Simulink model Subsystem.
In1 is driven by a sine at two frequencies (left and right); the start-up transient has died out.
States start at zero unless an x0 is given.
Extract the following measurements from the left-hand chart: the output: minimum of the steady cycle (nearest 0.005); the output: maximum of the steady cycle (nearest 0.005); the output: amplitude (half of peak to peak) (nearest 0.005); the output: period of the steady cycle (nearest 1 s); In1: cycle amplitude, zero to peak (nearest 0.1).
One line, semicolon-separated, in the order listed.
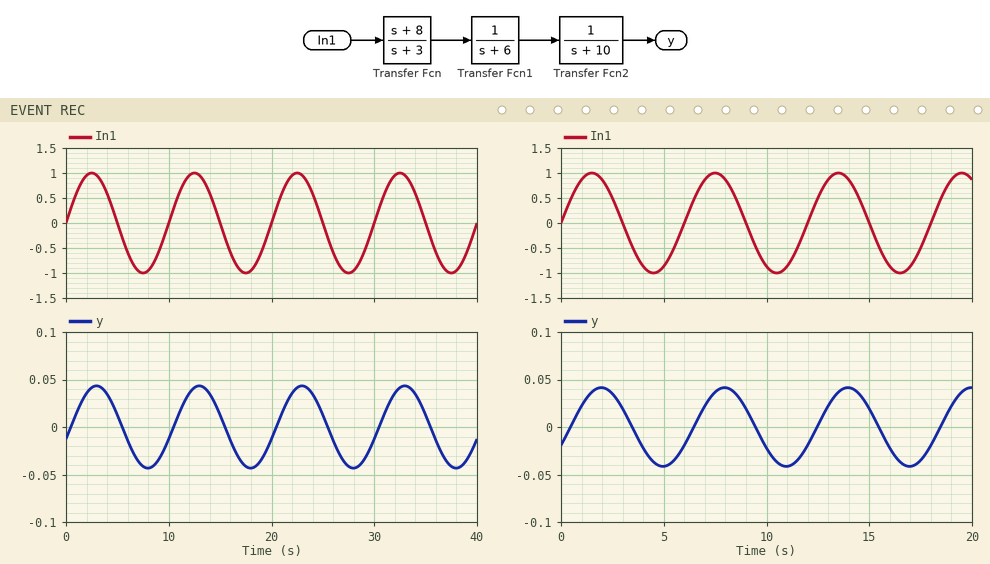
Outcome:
-0.045; 0.045; 0.045; 10 s; 1.0
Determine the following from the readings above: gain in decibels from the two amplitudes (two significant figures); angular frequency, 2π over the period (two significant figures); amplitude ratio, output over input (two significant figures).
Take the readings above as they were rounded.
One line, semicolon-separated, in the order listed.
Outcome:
-27 dB; 0.63 rad/s; 0.045
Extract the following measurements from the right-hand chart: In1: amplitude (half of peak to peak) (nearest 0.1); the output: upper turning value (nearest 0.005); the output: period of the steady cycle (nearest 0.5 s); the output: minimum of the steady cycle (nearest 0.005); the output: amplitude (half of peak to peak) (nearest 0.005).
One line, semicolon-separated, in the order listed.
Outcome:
1.0; 0.040; 6.0 s; -0.040; 0.040
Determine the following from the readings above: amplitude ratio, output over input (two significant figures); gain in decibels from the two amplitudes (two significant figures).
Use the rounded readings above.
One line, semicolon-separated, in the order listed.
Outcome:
0.040; -28 dB
